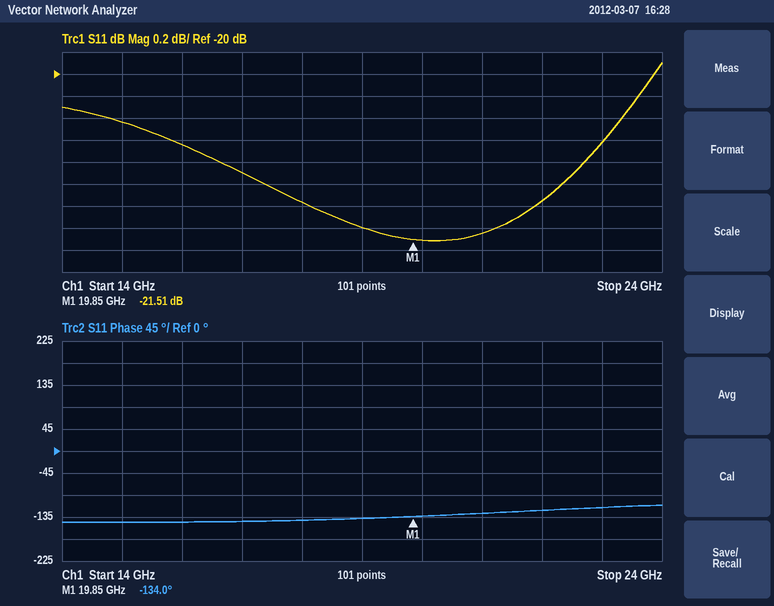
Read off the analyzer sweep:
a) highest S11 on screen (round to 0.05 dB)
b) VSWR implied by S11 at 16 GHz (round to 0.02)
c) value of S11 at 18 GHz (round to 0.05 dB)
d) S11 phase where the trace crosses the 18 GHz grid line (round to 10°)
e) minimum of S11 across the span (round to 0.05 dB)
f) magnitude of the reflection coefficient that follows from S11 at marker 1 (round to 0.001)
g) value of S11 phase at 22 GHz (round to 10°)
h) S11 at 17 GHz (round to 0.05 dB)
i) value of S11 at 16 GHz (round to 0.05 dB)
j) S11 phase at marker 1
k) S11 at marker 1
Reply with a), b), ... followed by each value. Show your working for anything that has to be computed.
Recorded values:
a) -19.90 dB
b) |Γ| = 10^(-20.65/20) = 0.0928; VSWR = (1 + 0.0928)/(1 − 0.0928) ≈ 1.20
c) -21.15 dB
d) -140°
e) -21.50 dB
f) 10^(-21.51/20) ≈ 0.084
g) -120°
h) -20.90 dB
i) -20.65 dB
j) -134.0°
k) -21.51 dB
